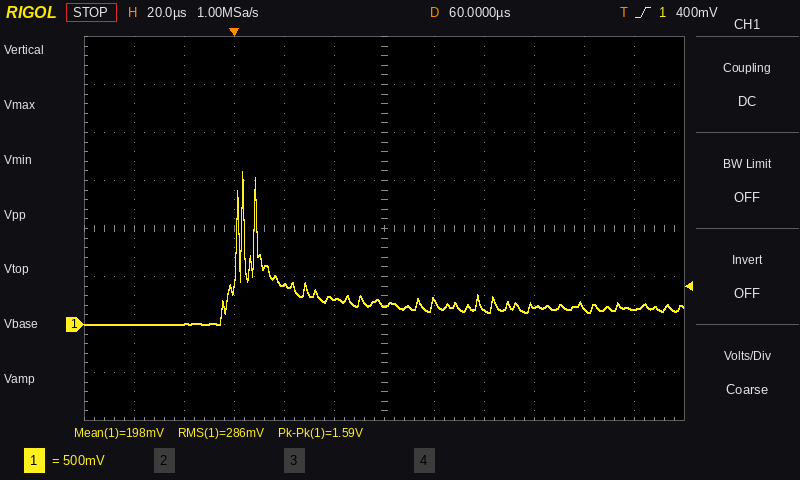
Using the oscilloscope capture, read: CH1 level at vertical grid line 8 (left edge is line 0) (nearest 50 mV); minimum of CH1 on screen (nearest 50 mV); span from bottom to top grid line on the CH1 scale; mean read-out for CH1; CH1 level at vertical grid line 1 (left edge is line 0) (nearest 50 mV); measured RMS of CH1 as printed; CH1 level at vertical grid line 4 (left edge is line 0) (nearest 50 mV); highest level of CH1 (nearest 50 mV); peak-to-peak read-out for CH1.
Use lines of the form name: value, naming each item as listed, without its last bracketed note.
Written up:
CH1 level at vertical grid line 8 (left edge is line 0): 150 mV
minimum of CH1 on screen: 0 mV
span from bottom to top grid line on the CH1 scale: 4 V
mean read-out for CH1: 198 mV
CH1 level at vertical grid line 1 (left edge is line 0): 0 mV
measured RMS of CH1 as printed: 286 mV
CH1 level at vertical grid line 4 (left edge is line 0): 400 mV
highest level of CH1: 1.60 V
peak-to-peak read-out for CH1: 1.59 V
